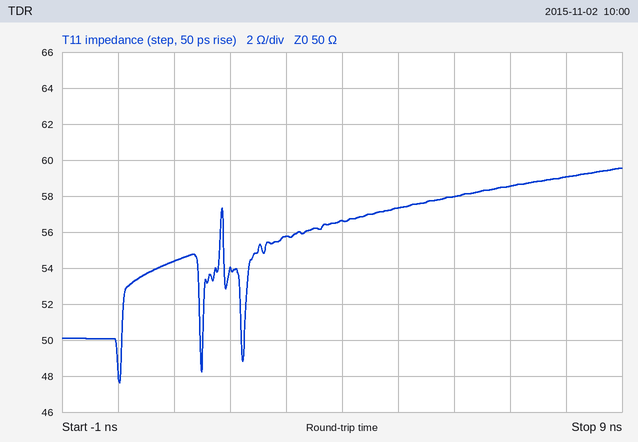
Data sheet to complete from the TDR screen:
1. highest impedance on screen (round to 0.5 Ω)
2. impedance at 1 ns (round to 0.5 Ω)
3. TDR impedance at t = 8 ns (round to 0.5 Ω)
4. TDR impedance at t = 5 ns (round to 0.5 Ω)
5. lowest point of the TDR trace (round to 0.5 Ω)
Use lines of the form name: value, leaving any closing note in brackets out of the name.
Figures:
highest impedance on screen: 59.5 Ω
impedance at 1 ns: 54.5 Ω
TDR impedance at t = 8 ns: 59.0 Ω
TDR impedance at t = 5 ns: 57.5 Ω
lowest point of the TDR trace: 47.5 Ω
